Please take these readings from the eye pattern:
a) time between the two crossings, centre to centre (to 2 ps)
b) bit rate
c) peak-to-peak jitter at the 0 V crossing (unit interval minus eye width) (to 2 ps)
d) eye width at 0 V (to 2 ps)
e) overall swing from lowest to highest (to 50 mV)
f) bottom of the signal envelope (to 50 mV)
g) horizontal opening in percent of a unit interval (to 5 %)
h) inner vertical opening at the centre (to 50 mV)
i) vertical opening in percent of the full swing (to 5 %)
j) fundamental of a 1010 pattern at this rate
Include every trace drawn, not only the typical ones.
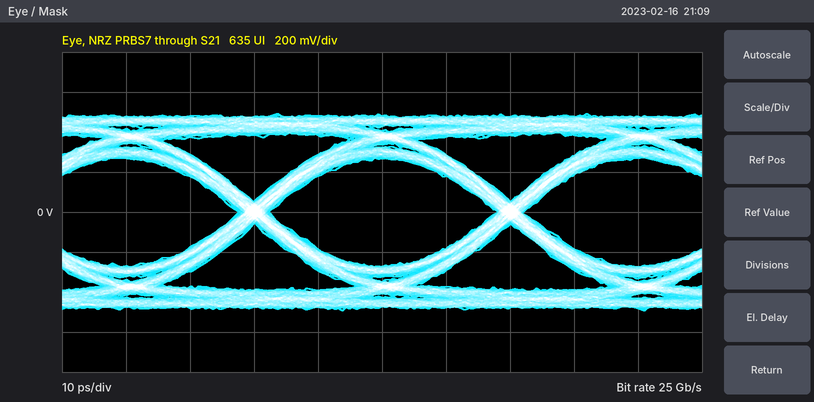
40 ps
25 Gb/s
4 ps
36 ps
1.00 V
-500 mV
90 %
550 mV
55 %
12.5 GHz
